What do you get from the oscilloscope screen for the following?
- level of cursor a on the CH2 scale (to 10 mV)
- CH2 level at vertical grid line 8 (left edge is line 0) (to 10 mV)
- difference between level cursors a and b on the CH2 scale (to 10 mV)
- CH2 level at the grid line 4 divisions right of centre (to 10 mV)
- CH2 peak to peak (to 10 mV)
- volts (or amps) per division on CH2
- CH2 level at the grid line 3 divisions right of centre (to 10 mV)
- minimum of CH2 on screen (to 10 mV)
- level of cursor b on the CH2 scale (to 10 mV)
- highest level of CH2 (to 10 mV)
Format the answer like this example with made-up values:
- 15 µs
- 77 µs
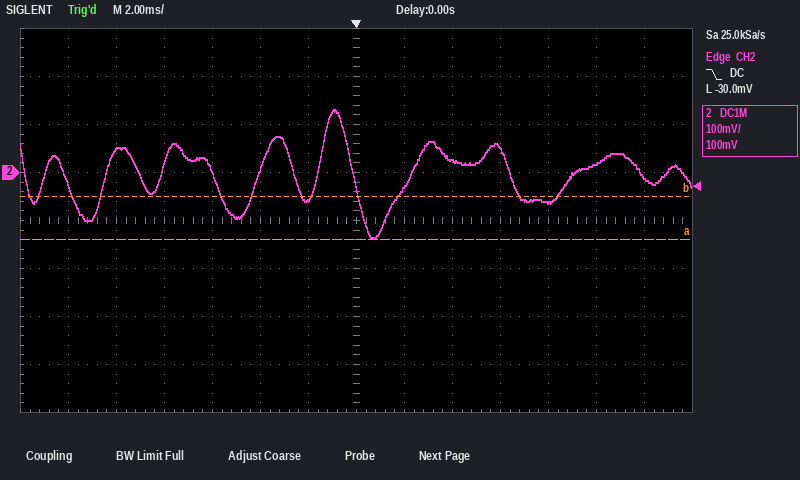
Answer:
- -140 mV
- -30 mV
- 90 mV
- -60 mV
- 270 mV
- 100 mV
- 50 mV
- -140 mV
- -50 mV
- 130 mV
